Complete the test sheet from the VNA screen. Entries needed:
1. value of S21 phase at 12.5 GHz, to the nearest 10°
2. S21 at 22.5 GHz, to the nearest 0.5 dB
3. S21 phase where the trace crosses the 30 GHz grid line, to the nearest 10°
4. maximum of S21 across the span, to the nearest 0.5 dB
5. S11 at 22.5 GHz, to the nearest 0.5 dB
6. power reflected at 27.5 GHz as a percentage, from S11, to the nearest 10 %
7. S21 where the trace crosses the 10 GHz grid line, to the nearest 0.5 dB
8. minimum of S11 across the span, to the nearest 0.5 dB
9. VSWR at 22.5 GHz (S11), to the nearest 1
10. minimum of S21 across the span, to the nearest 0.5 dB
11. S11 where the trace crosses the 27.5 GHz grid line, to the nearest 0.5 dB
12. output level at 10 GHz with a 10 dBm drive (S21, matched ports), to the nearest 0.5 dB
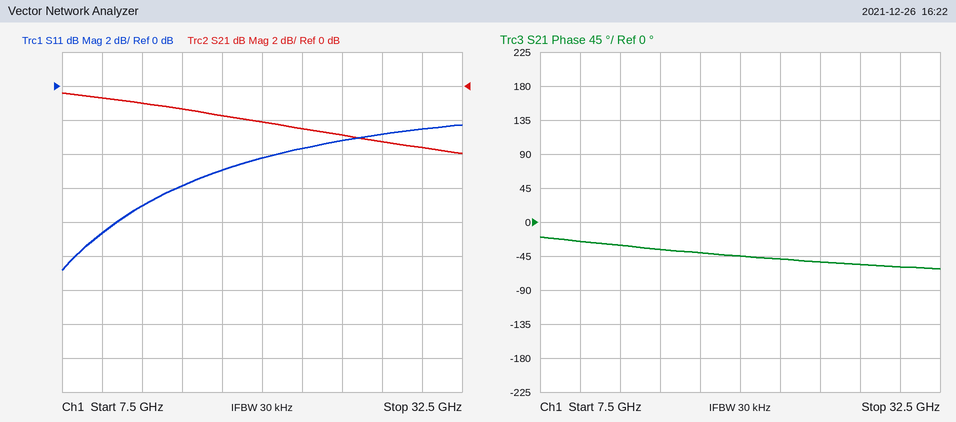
-30°
-2.5 dB
-60°
-0.5 dB
-3.5 dB
50 %
-0.5 dB
-11.0 dB
5
-4.0 dB
-3.0 dB
9.5 dBm
